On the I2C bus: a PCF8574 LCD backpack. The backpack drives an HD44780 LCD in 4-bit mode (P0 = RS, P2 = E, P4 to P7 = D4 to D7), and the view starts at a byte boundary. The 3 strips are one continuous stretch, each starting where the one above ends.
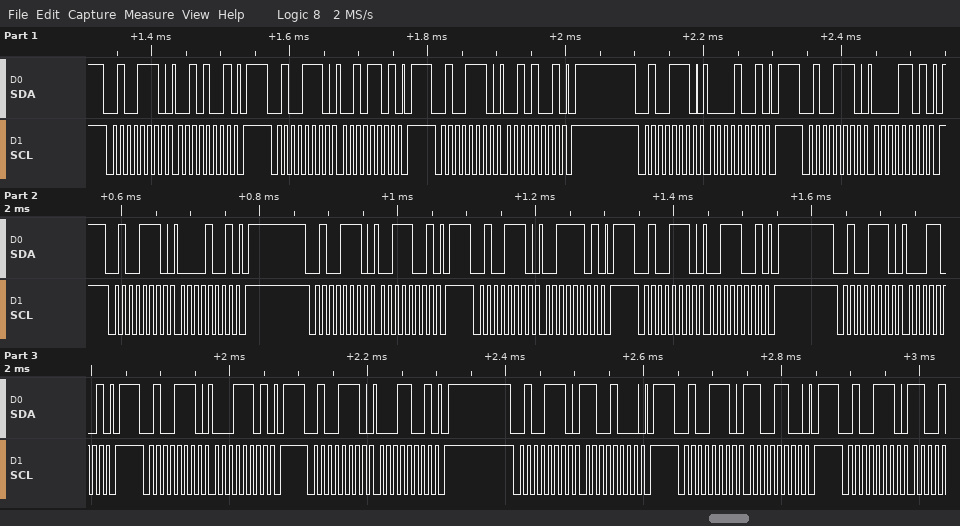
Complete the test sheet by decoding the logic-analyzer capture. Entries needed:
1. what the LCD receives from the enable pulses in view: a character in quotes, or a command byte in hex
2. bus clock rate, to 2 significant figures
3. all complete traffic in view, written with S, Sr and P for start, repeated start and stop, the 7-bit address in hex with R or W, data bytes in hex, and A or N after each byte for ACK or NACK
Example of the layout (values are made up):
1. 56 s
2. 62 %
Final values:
1. ' ' '1'
2. 100 kHz
3. S 27W A 29 A P S 27W A 2D A P S 27W A 29 A P S 27W A 09 A P S 27W A 0D A P S 27W A 09 A P S 27W A 39 A P S 27W A 3D A P S 27W A 39 A P S 27W A 19 A P S 27W A 1D A P S 27W A 19 A P S 27W A C8 A P S 27W A CC A P S 27W A
